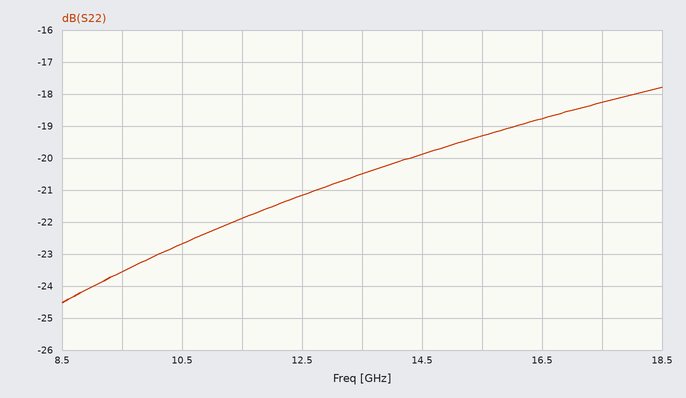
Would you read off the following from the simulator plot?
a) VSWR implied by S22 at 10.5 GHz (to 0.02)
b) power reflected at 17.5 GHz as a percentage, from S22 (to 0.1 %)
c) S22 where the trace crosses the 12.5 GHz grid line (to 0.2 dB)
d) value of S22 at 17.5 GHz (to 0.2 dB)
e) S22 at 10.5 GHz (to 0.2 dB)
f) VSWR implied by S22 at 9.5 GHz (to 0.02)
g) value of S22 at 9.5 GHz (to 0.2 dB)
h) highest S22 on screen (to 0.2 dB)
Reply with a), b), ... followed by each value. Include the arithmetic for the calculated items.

a) |Γ| = 10^(-22.6/20) = 0.0741; VSWR = (1 + 0.0741)/(1 − 0.0741) ≈ 1.16
b) 10^(-18.2/10) ≈ 1.5 %
c) -21.2 dB
d) -18.2 dB
e) -22.6 dB
f) |Γ| = 10^(-23.6/20) = 0.0661; VSWR = (1 + 0.0661)/(1 − 0.0661) ≈ 1.14
g) -23.6 dB
h) -17.8 dB
